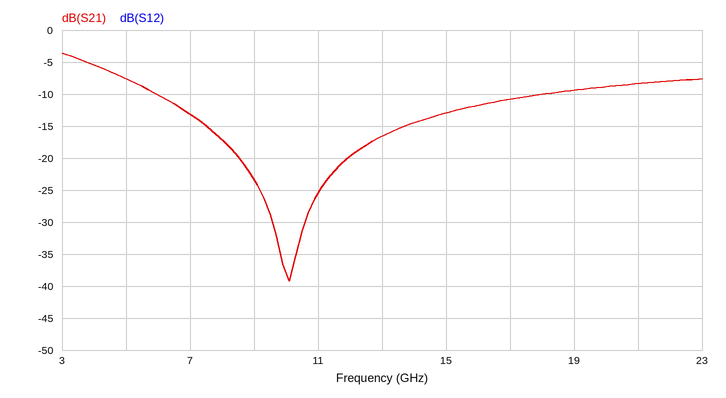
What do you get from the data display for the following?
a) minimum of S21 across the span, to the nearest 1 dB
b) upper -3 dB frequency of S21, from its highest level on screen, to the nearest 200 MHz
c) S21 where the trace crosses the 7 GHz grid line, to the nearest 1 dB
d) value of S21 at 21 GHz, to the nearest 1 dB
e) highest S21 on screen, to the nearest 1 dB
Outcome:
-39 dB
4.6 GHz
-13 dB
-8 dB
-4 dB
